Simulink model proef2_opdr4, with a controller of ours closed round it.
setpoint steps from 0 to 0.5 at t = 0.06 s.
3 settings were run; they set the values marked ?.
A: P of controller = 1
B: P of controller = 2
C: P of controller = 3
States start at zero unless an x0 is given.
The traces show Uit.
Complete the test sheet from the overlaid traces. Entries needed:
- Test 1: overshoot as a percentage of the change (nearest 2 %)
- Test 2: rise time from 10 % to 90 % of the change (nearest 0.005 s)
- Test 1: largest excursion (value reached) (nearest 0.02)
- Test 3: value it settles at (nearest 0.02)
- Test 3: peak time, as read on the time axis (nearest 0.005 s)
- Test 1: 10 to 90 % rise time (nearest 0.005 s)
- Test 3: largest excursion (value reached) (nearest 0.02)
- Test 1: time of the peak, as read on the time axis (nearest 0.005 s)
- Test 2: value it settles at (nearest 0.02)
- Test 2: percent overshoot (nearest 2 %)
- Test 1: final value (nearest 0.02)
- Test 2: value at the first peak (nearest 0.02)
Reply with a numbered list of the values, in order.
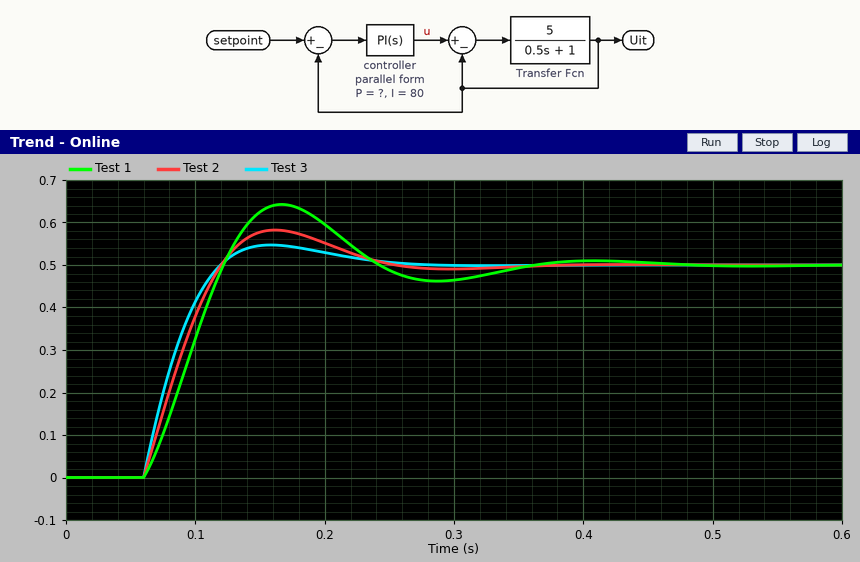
1. 28 %
2. 0.045 s
3. 0.64
4. 0.50
5. 0.160 s
6. 0.045 s
7. 0.54
8. 0.165 s
9. 0.50
10. 16 %
11. 0.50
12. 0.58
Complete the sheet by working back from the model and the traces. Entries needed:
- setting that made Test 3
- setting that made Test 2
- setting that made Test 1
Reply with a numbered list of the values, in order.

1. C
2. B
3. A
